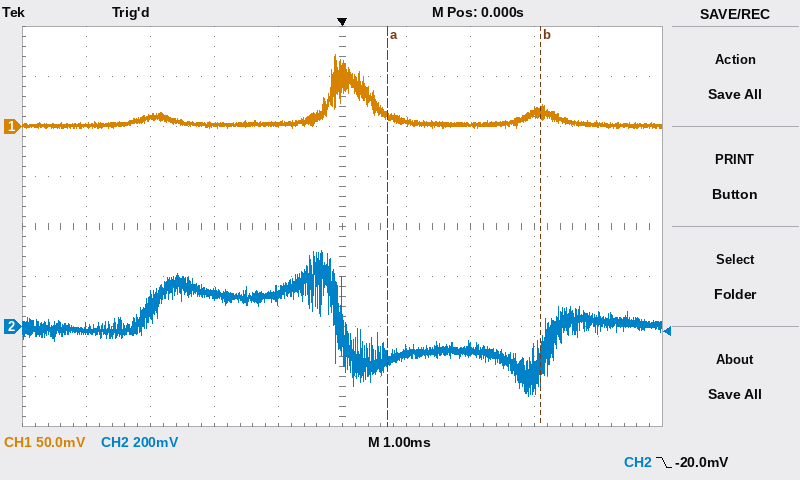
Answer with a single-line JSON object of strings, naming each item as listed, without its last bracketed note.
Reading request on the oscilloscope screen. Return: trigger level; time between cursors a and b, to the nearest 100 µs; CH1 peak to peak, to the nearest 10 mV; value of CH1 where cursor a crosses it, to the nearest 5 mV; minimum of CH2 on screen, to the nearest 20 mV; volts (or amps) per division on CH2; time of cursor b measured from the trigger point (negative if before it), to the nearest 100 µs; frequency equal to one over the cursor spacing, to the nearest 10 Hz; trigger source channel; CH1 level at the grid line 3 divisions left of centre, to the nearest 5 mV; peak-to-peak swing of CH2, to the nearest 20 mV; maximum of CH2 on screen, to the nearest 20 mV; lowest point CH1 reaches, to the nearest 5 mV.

{"trigger level": "-20.0 mV", "time between cursors a and b, to the nearest 100 µs": "2.4 ms", "CH1 peak to peak, to the nearest 10 mV": "70 mV", "value of CH1 where cursor a crosses it, to the nearest 5 mV": "10 mV", "minimum of CH2 on screen, to the nearest 20 mV": "-280 mV", "volts (or amps) per division on CH2": "200 mV", "time of cursor b measured from the trigger point (negative if before it), to the nearest 100 µs": "+3.1 ms", "frequency equal to one over the cursor spacing, to the nearest 10 Hz": "420 Hz", "trigger source channel": "CH2", "CH1 level at the grid line 3 divisions left of centre, to the nearest 5 mV": "10 mV", "peak-to-peak swing of CH2, to the nearest 20 mV": "580 mV", "maximum of CH2 on screen, to the nearest 20 mV": "300 mV", "lowest point CH1 reaches, to the nearest 5 mV": "0 mV"}
